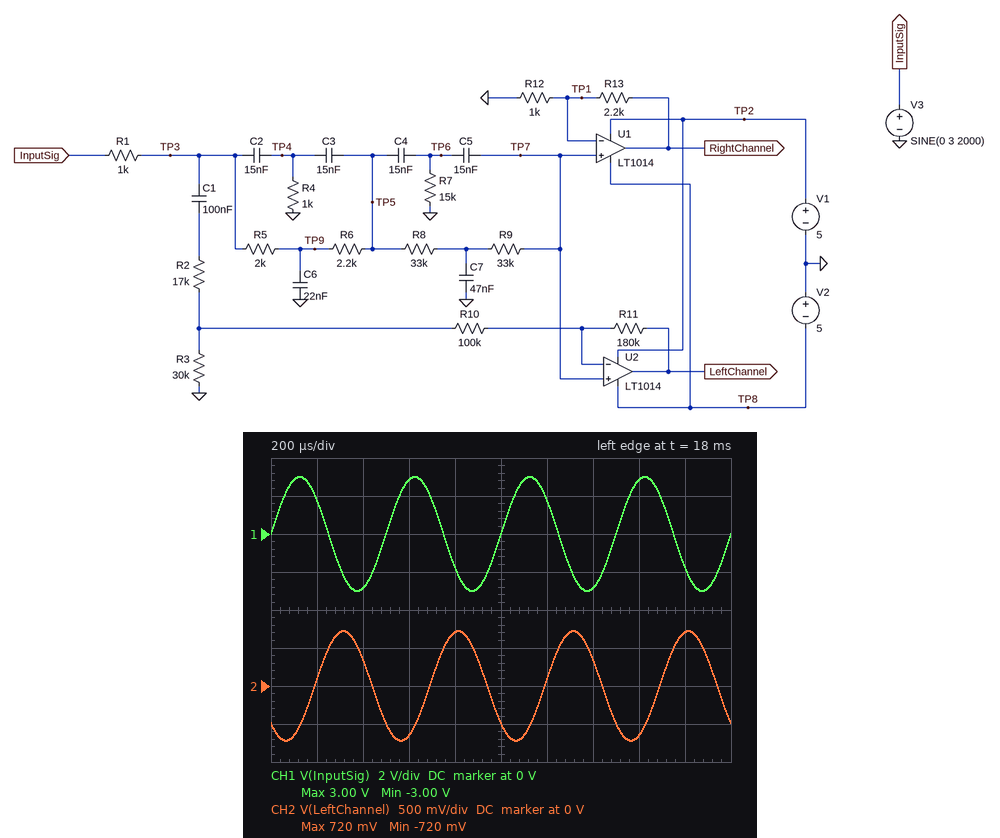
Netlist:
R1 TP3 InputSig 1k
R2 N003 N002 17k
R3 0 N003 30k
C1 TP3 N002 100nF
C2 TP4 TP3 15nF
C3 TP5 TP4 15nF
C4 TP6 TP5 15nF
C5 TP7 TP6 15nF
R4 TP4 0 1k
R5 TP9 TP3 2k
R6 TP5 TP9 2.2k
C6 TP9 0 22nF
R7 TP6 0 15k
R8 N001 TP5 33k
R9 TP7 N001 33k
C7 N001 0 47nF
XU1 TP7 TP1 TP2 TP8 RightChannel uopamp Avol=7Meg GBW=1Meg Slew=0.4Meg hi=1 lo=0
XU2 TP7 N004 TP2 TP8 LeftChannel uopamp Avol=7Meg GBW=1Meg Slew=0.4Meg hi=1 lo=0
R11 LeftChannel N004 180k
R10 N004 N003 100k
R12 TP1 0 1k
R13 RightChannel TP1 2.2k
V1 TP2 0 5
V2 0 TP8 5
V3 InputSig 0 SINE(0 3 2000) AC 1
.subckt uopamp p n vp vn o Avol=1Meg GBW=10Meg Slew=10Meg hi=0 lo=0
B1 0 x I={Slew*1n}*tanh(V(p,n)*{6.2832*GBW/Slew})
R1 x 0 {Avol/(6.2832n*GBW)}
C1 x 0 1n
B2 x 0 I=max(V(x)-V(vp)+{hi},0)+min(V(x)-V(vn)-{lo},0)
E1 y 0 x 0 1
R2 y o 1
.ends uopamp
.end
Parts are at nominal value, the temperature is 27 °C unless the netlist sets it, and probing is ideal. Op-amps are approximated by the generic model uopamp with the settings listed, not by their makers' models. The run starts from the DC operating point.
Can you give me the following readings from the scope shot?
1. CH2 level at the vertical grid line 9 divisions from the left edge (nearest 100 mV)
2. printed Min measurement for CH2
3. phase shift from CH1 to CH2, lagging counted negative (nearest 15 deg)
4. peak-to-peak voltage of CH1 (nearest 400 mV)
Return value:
700 mV
-720 mV
-135 deg
6.0 V
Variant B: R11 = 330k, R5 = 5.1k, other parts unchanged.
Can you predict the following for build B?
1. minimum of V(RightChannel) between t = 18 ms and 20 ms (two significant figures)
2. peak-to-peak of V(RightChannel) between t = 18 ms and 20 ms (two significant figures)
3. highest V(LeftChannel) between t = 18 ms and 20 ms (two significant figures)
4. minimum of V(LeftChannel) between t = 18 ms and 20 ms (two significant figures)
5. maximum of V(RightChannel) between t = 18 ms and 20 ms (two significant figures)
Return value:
-1.3 V
2.6 V
3.5 V
-3.5 V
1.3 V
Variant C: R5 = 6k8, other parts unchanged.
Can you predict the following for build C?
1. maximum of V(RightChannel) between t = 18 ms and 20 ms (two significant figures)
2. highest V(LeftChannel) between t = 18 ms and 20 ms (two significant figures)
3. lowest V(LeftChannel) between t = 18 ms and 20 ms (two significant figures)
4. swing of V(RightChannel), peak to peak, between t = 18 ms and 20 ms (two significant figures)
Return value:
990 mV
2.1 V
-2.1 V
2.0 V
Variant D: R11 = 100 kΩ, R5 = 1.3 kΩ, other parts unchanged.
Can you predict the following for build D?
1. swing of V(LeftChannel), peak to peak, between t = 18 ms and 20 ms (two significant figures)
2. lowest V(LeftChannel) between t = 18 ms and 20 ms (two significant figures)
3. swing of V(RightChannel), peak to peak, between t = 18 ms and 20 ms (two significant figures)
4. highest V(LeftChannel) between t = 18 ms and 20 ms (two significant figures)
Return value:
1.0 V
-520 mV
5.9 V
520 mV
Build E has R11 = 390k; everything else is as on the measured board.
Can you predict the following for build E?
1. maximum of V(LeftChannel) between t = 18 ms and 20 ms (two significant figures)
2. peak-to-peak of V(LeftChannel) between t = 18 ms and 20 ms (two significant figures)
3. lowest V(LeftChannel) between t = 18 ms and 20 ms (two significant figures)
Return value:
2.0 V
4.0 V
-2.0 V
